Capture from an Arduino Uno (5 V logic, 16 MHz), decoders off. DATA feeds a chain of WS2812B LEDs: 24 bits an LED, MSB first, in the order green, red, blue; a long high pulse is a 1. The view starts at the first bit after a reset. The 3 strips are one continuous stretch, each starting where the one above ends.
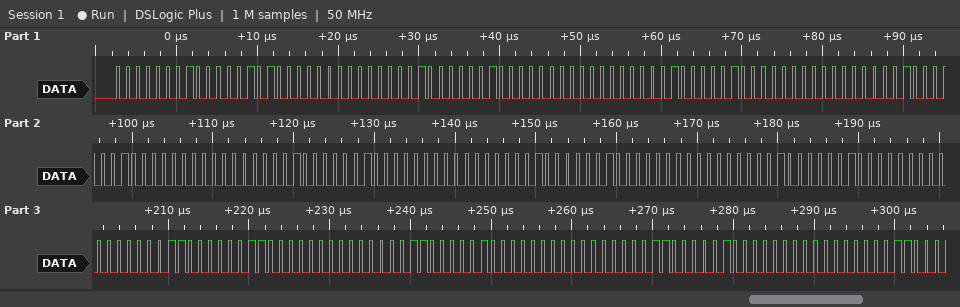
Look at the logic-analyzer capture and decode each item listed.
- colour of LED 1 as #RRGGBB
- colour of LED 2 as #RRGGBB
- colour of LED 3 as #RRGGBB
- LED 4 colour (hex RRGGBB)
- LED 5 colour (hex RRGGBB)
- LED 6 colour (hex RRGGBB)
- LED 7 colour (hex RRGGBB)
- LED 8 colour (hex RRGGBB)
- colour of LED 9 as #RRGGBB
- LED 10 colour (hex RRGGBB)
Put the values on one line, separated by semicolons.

#050100; #040200; #040100; #040200; #040200; #040200; #040200; #030300; #040300; #040300
